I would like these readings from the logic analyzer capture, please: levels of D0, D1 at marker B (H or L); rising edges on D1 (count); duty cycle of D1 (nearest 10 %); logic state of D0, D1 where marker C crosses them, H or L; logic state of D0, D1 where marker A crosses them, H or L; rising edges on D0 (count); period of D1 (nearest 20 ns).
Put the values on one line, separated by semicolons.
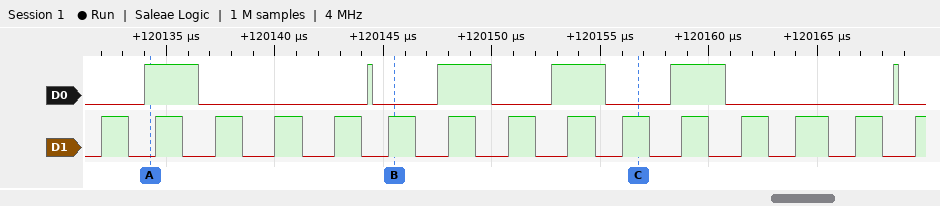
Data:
D0=L, D1=H; 15; 50 %; D0=L, D1=H; D0=H, D1=L; 6; 2680 ns
